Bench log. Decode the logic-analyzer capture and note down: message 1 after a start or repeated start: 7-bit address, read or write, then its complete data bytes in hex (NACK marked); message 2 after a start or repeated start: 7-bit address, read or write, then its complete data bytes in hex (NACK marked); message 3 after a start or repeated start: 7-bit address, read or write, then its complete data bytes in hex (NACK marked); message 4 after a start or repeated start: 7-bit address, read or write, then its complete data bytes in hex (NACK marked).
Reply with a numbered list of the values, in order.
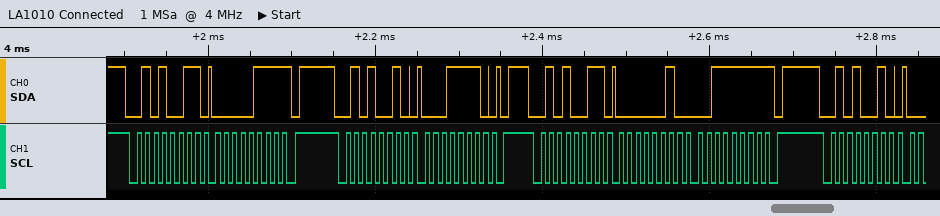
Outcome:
1. 0x29 read: 07 NACK
2. 0x29 write: 1E
3. 0x29 read: 02 3F NACK
4. 0x29 write
